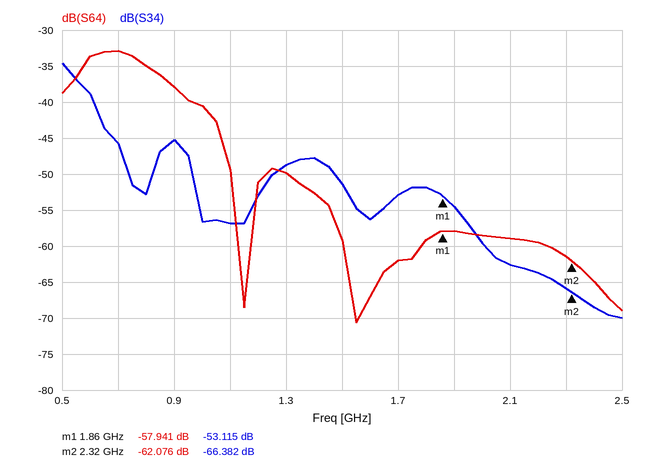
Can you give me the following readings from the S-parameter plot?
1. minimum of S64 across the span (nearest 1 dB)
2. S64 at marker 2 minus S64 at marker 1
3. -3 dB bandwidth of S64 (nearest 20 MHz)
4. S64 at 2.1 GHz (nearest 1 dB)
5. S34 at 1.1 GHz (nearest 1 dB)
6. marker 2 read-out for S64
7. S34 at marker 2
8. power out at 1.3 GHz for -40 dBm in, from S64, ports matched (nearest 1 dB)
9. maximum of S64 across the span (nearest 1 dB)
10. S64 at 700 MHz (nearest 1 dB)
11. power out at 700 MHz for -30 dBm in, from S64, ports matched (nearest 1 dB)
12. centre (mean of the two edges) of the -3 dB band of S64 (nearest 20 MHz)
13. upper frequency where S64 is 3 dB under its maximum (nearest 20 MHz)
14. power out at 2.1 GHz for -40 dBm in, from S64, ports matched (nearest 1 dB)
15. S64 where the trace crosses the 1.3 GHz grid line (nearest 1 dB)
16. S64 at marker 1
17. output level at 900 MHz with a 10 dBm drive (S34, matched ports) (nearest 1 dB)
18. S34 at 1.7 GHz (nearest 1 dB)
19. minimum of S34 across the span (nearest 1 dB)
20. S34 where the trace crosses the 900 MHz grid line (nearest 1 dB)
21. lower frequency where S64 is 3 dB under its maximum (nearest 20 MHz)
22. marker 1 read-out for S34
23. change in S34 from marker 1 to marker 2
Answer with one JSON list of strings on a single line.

["-71 dB", "-4.135 dB", "280 MHz", "-59 dB", "-57 dB", "-62.076 dB", "-66.382 dB", "-90 dBm", "-33 dB", "-33 dB", "-63 dBm", "700 MHz", "840 MHz", "-99 dBm", "-50 dB", "-57.941 dB", "-35 dBm", "-53 dB", "-70 dB", "-45 dB", "560 MHz", "-53.115 dB", "-13.267 dB"]
